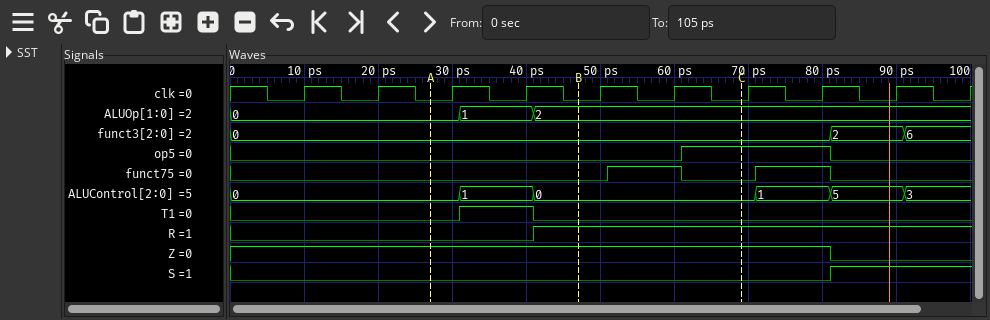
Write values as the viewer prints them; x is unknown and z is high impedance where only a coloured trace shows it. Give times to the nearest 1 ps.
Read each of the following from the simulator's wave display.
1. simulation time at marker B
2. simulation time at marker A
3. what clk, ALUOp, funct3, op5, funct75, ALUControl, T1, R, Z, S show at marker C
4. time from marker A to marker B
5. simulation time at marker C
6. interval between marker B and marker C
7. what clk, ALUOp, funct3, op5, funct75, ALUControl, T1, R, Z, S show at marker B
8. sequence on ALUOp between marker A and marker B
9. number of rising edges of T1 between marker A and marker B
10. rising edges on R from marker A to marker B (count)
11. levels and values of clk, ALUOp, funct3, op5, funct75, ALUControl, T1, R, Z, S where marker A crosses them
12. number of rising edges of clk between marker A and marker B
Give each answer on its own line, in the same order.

47 ps
27 ps
clk=0, ALUOp=2, funct3=0, op5=1, funct75=0, ALUControl=0, T1=0, R=1, Z=1, S=0
20 ps
69 ps
22 ps
clk=0, ALUOp=2, funct3=0, op5=0, funct75=0, ALUControl=0, T1=0, R=1, Z=1, S=0
0, 1, 2
1
1
clk=0, ALUOp=0, funct3=0, op5=0, funct75=0, ALUControl=0, T1=0, R=0, Z=1, S=0
2
